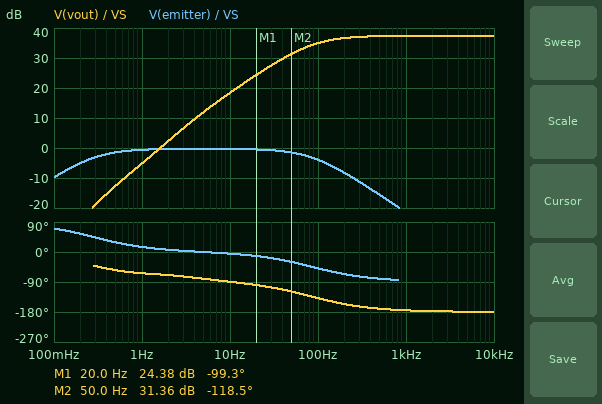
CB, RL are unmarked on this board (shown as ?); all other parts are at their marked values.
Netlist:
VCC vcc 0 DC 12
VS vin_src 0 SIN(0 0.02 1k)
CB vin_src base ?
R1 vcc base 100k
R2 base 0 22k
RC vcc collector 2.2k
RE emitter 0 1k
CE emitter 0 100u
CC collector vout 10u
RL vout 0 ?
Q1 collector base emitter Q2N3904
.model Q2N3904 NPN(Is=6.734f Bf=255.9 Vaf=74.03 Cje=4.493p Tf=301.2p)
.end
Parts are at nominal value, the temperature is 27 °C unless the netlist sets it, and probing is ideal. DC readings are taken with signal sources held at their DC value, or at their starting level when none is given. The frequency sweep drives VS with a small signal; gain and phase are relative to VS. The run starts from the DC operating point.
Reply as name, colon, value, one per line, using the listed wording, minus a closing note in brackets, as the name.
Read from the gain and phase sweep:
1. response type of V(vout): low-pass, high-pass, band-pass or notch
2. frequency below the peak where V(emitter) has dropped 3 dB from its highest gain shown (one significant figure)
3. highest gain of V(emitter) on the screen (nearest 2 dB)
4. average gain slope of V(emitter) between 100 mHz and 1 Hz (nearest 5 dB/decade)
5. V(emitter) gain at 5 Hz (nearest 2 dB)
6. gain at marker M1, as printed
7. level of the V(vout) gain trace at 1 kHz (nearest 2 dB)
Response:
response type of V(vout): low-pass, high-pass, band-pass or notch: high-pass
frequency below the peak where V(emitter) has dropped 3 dB from its highest gain shown: 300 mHz
highest gain of V(emitter) on the screen: 0 dB
average gain slope of V(emitter) between 100 mHz and 1 Hz: 10 dB/decade
V(emitter) gain at 5 Hz: 0 dB
gain at marker M1, as printed: 24.38 dB
level of the V(vout) gain trace at 1 kHz: 38 dB
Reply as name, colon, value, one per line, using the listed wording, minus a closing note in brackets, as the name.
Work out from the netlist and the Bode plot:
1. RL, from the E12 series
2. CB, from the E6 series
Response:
RL, from the E12 series: 3.9 kΩ
CB, from the E6 series: 33 µF
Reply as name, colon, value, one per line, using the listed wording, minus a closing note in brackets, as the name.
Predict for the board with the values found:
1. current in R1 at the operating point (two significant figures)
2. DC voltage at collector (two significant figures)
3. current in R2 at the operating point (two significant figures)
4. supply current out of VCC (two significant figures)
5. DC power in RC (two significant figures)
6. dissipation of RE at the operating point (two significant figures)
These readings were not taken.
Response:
current in R1 at the operating point: 99 µA
DC voltage at collector: 8.9 V
current in R2 at the operating point: 94 µA
supply current out of VCC: 1.5 mA
DC power in RC: 4.3 mW
dissipation of RE at the operating point: 2.0 mW
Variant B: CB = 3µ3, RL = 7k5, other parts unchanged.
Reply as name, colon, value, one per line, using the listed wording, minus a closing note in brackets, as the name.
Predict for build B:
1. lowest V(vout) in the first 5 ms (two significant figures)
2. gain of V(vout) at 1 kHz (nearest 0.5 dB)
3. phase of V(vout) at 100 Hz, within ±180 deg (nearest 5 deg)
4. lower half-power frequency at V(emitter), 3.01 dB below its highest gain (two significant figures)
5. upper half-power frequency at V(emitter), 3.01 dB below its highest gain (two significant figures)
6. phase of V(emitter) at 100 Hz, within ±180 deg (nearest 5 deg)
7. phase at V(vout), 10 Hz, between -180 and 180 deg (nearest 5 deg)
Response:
lowest V(vout) in the first 5 ms: -2.2 V
gain of V(vout) at 1 kHz: 39.0 dB
phase of V(vout) at 100 Hz, within ±180 deg: -135 deg
lower half-power frequency at V(emitter), 3.01 dB below its highest gain: 2.4 Hz
upper half-power frequency at V(emitter), 3.01 dB below its highest gain: 100 Hz
phase of V(emitter) at 100 Hz, within ±180 deg: -45 deg
phase at V(vout), 10 Hz, between -180 and 180 deg: -80 deg
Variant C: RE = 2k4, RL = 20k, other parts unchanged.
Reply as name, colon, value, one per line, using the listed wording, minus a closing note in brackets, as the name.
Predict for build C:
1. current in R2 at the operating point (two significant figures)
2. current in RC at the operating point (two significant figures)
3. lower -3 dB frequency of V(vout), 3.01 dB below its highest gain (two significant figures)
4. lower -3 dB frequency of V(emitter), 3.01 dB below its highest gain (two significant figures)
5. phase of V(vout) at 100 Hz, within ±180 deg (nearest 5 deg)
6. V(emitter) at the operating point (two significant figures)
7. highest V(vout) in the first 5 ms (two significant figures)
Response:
current in R2 at the operating point: 97 µA
current in RC at the operating point: 610 µA
lower -3 dB frequency of V(vout), 3.01 dB below its highest gain: 38 Hz
lower -3 dB frequency of V(emitter), 3.01 dB below its highest gain: 270 mHz
phase of V(vout) at 100 Hz, within ±180 deg: -160 deg
V(emitter) at the operating point: 1.5 V
highest V(vout) in the first 5 ms: 710 mV
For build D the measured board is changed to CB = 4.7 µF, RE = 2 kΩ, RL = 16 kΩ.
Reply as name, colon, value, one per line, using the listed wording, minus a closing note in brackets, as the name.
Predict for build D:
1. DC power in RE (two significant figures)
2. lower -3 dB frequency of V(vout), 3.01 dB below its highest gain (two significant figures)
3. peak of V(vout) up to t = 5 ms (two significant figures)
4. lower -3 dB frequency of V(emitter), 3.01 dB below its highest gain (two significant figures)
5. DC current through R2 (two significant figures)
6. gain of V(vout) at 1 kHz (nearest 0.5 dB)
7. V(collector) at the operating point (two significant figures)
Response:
DC power in RE: 1.1 mW
lower -3 dB frequency of V(vout), 3.01 dB below its highest gain: 49 Hz
peak of V(vout) up to t = 5 ms: 830 mV
lower -3 dB frequency of V(emitter), 3.01 dB below its highest gain: 1.7 Hz
DC current through R2: 96 µA
gain of V(vout) at 1 kHz: 34.5 dB
V(collector) at the operating point: 10 V
